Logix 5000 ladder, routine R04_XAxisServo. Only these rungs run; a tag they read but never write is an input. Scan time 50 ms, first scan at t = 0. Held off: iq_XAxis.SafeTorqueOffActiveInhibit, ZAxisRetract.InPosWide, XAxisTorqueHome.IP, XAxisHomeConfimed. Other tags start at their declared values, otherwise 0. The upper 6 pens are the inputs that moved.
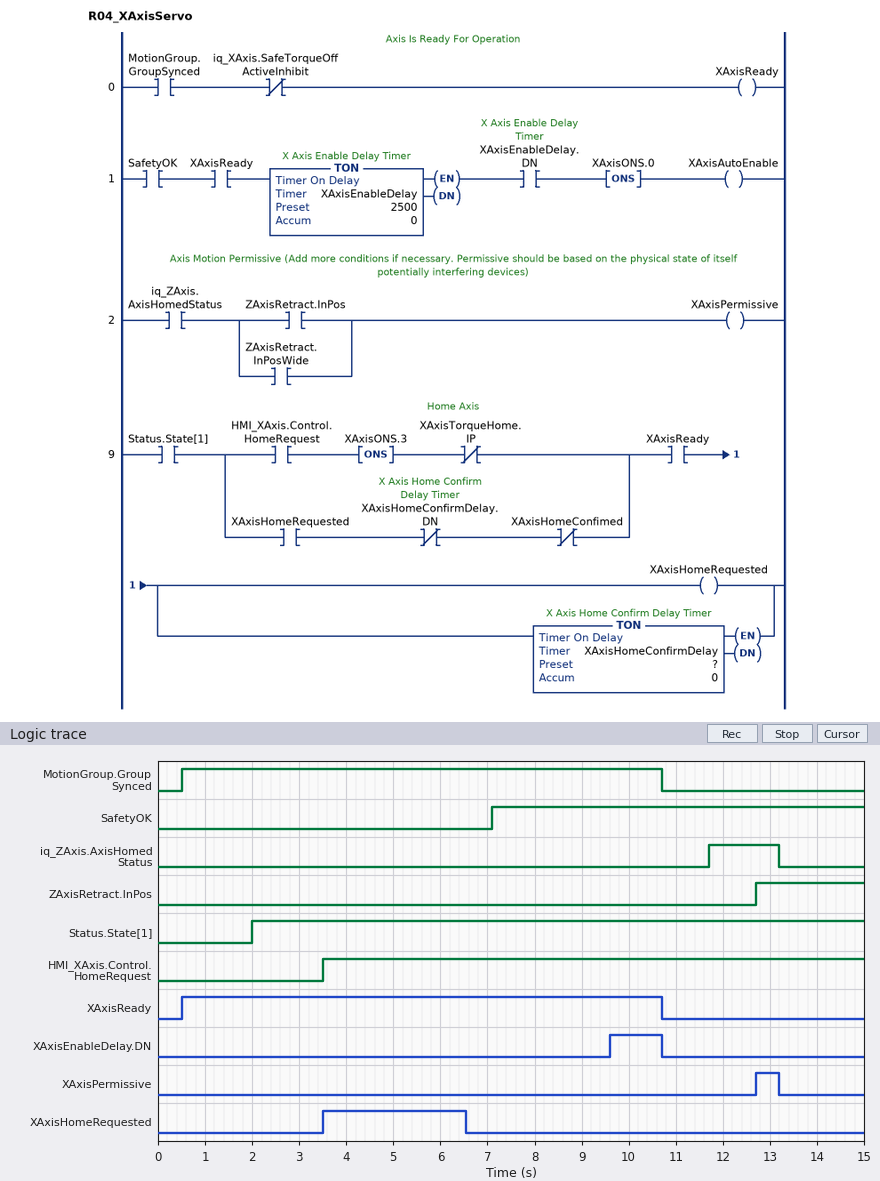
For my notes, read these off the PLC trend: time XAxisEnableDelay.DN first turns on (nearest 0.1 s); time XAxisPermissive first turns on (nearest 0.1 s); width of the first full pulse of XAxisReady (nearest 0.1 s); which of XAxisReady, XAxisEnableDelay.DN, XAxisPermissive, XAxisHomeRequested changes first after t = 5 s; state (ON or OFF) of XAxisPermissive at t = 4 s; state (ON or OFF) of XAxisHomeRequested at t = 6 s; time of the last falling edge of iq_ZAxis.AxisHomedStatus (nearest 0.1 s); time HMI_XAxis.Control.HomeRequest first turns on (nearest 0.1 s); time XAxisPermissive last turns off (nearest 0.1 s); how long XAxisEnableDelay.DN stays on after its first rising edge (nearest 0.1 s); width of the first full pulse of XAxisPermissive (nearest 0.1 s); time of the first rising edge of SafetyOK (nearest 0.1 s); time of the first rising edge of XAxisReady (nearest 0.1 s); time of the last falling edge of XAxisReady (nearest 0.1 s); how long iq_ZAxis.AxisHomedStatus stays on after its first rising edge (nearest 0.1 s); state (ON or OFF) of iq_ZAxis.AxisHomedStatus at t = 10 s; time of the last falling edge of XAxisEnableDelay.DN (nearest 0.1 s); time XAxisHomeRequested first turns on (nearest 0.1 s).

9.6 s
12.7 s
10.2 s
XAxisHomeRequested
OFF
ON
13.2 s
3.5 s
13.2 s
1.1 s
0.5 s
7.1 s
0.5 s
10.7 s
1.5 s
OFF
10.7 s
3.5 s
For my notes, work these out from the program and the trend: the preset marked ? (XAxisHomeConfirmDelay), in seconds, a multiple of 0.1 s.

3.0 s
